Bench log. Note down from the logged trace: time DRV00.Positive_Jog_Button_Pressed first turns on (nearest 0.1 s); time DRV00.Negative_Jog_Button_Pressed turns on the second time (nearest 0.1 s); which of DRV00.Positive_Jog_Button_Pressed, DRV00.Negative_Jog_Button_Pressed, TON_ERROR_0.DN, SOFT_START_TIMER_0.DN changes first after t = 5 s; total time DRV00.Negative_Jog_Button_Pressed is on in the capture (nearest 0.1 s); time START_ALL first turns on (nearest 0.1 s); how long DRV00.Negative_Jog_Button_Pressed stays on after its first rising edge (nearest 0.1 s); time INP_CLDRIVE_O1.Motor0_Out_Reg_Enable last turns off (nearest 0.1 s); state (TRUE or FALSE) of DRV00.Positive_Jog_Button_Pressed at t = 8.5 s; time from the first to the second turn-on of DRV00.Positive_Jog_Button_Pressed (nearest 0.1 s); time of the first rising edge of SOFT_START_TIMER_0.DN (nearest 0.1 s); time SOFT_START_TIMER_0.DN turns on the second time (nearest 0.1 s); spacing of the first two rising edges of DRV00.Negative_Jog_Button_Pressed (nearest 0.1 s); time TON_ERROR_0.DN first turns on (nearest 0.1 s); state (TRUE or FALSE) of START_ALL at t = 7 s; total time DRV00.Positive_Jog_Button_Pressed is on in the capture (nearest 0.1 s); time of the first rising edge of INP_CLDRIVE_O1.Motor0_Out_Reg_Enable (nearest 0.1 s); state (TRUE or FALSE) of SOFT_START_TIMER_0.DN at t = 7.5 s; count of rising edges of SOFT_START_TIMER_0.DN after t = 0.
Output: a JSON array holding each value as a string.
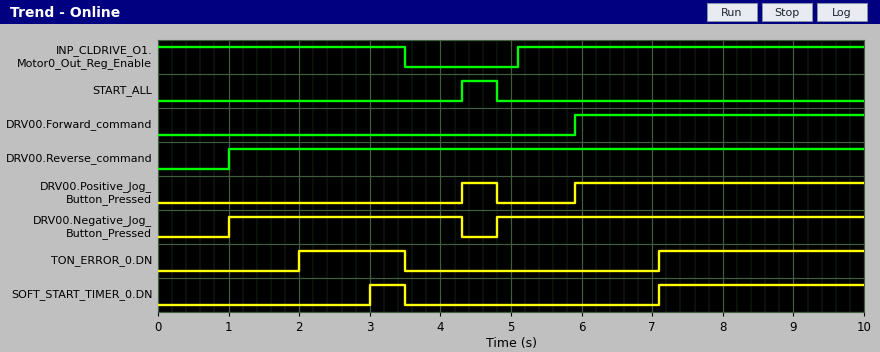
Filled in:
["4.3 s", "4.8 s", "DRV00.Positive_Jog_Button_Pressed", "8.5 s", "4.3 s", "3.3 s", "3.5 s", "TRUE", "1.6 s", "3.0 s", "7.1 s", "3.8 s", "2.0 s", "FALSE", "4.6 s", "5.1 s", "TRUE", "2"]
